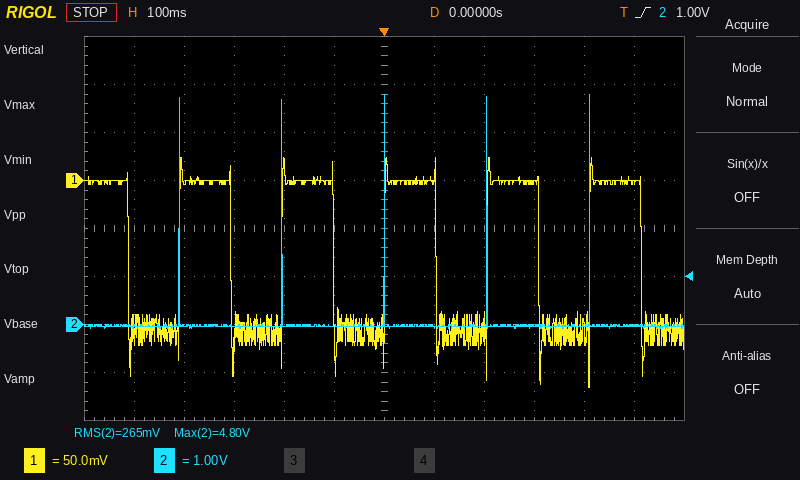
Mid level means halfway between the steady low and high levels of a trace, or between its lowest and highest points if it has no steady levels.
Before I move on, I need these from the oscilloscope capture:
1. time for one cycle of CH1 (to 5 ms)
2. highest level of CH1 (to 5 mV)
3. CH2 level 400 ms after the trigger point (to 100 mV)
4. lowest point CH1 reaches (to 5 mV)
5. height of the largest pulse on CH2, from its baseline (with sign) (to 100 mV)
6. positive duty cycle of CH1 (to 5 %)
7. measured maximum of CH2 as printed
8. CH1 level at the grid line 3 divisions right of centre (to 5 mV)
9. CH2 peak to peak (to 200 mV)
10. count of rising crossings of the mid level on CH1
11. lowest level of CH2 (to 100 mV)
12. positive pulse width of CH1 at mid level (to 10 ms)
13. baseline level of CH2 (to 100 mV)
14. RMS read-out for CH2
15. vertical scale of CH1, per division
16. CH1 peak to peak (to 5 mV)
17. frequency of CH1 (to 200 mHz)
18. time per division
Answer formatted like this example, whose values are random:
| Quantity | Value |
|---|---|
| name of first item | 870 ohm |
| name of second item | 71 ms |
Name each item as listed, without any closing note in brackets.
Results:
| Quantity | Value |
|---|---|
| time for one cycle of CH1 | 205 ms |
| highest level of CH1 | 25 mV |
| CH2 level 400 ms after the trigger point | 0.0 V |
| lowest point CH1 reaches | -215 mV |
| height of the largest pulse on CH2, from its baseline (with sign) | +4.8 V |
| positive duty cycle of CH1 | 50 % |
| measured maximum of CH2 as printed | 4.80 V |
| CH1 level at the grid line 3 divisions right of centre | 0 mV |
| CH2 peak to peak | 4.8 V |
| count of rising crossings of the mid level on CH1 | 5 |
| lowest level of CH2 | -100 mV |
| positive pulse width of CH1 at mid level | 100 ms |
| baseline level of CH2 | 0.0 V |
| RMS read-out for CH2 | 265 mV |
| vertical scale of CH1, per division | 50 mV |
| CH1 peak to peak | 240 mV |
| frequency of CH1 | 4.8 Hz |
| time per division | 100 ms |
